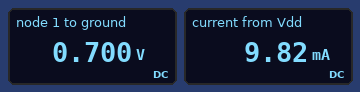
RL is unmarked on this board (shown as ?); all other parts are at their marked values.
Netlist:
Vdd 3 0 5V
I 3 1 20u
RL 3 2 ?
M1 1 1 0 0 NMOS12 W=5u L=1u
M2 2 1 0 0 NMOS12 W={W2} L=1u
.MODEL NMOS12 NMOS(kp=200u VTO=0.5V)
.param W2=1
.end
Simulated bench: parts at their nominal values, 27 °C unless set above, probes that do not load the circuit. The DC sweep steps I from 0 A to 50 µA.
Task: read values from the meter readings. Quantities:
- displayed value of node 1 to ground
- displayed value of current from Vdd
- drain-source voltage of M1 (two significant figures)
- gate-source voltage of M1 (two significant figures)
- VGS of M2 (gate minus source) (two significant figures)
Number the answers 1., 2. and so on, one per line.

1. 0.700 V
2. 9.82 mA
3. 700 mV
4. 700 mV
5. 700 mV
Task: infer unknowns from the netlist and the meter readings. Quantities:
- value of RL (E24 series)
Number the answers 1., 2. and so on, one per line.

1. 510 Ω
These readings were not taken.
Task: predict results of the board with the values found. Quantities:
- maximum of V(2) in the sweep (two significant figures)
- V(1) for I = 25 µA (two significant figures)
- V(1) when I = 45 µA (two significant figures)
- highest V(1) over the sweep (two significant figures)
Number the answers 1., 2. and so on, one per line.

1. 5.0 V
2. 720 mV
3. 800 mV
4. 820 mV
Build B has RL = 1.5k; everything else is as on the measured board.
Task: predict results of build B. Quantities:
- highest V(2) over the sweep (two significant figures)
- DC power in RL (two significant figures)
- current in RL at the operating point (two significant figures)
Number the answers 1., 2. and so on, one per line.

1. 5.0 V
2. 17 mW
3. 3.3 mA
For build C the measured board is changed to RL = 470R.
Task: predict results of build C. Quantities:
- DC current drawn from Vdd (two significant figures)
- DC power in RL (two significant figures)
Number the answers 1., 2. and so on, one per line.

1. 11 mA
2. 53 mW
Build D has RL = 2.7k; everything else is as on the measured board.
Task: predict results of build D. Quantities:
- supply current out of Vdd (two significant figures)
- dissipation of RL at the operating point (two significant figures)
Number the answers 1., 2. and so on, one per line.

1. 1.9 mA
2. 9.3 mW
